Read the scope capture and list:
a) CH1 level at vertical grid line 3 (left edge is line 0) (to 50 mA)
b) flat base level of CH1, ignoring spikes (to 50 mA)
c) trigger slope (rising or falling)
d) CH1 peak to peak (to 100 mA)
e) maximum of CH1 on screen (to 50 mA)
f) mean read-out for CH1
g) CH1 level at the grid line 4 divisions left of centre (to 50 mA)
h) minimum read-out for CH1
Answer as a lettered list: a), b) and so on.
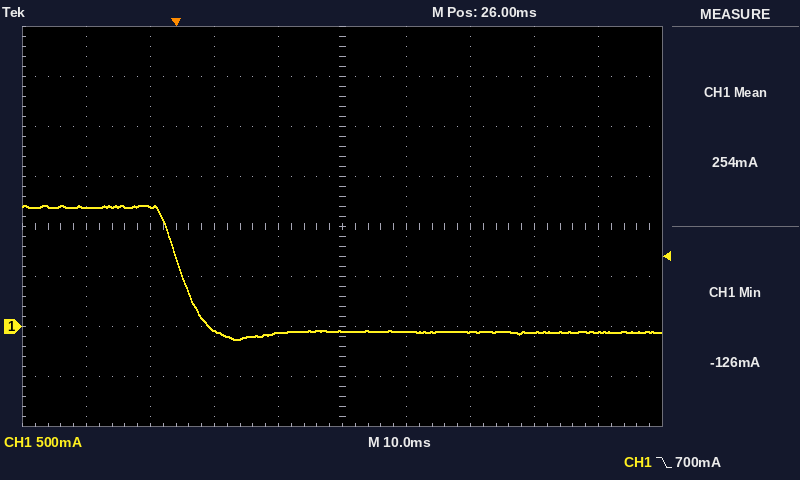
a) -50 mA
b) -50 mA
c) falling
d) 1.30 A
e) 1.20 A
f) 254 mA
g) 1.20 A
h) -126 mA
